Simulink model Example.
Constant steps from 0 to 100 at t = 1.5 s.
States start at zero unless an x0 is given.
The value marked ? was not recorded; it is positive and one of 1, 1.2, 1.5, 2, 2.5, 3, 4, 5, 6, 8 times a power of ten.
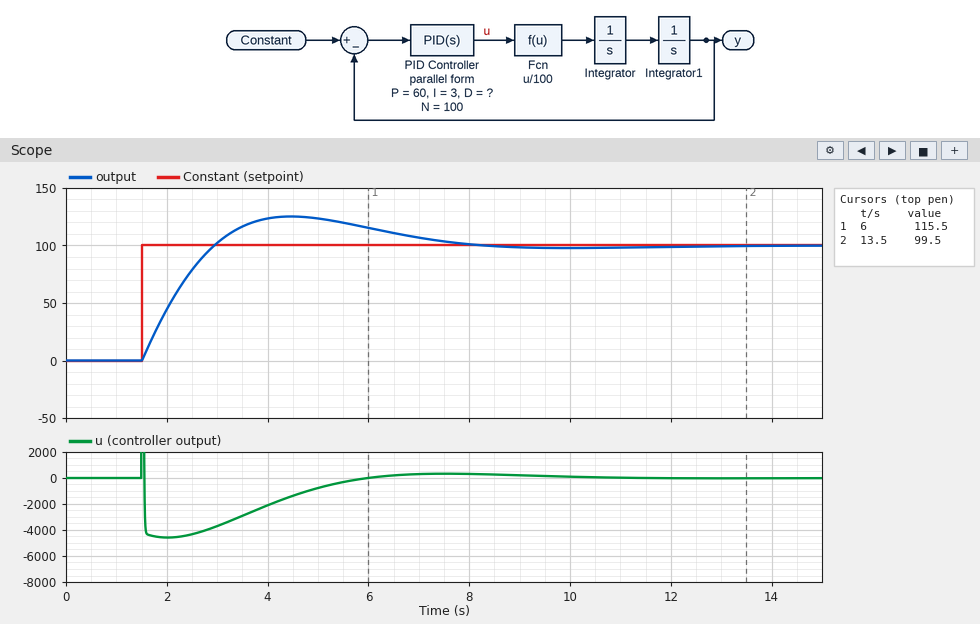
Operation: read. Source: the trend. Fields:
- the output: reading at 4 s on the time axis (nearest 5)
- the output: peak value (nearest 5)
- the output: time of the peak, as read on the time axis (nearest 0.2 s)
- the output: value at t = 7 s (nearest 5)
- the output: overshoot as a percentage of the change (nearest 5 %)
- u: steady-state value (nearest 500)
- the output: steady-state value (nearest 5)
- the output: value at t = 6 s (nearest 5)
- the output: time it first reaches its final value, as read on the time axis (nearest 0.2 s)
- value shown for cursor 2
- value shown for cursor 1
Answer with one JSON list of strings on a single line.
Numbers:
["125", "125", "4.4 s", "105", "25 %", "0", "100", "115", "3.0 s", "99.5", "115.5"]
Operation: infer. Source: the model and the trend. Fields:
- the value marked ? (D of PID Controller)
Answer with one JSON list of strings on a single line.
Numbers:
["100"]
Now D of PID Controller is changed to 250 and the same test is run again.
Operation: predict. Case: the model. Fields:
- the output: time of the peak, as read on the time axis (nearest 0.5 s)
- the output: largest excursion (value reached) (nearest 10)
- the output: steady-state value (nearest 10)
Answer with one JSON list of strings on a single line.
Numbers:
["3.5 s", "110", "100"]
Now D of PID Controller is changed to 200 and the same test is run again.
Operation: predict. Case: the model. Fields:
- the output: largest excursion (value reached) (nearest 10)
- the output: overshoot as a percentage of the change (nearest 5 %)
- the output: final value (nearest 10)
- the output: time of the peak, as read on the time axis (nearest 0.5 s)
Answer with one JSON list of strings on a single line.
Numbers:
["110", "10 %", "100", "4.0 s"]
